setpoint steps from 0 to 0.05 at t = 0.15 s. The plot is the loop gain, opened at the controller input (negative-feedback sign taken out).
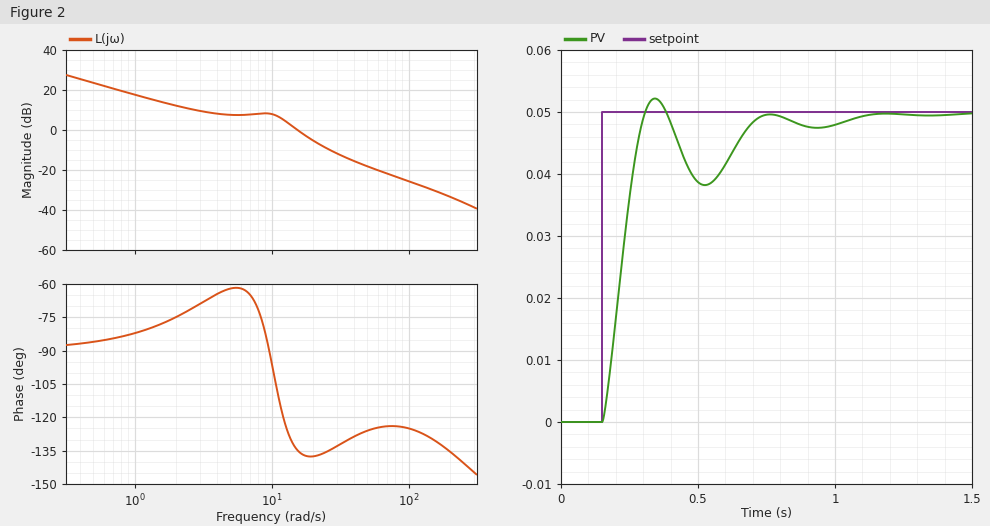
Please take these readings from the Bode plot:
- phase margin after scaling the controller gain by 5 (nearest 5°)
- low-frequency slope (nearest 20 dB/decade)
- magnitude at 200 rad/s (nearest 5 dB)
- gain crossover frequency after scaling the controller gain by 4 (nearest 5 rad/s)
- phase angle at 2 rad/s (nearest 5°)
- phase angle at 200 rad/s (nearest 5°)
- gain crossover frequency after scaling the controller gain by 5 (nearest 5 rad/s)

50°
-20 dB/decade
-35 dB
30 rad/s
-75°
-135°
35 rad/s
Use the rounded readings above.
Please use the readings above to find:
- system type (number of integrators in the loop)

1
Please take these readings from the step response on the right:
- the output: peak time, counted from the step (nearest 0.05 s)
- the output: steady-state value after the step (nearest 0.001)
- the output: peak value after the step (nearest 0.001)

0.20 s
0.050
0.052
